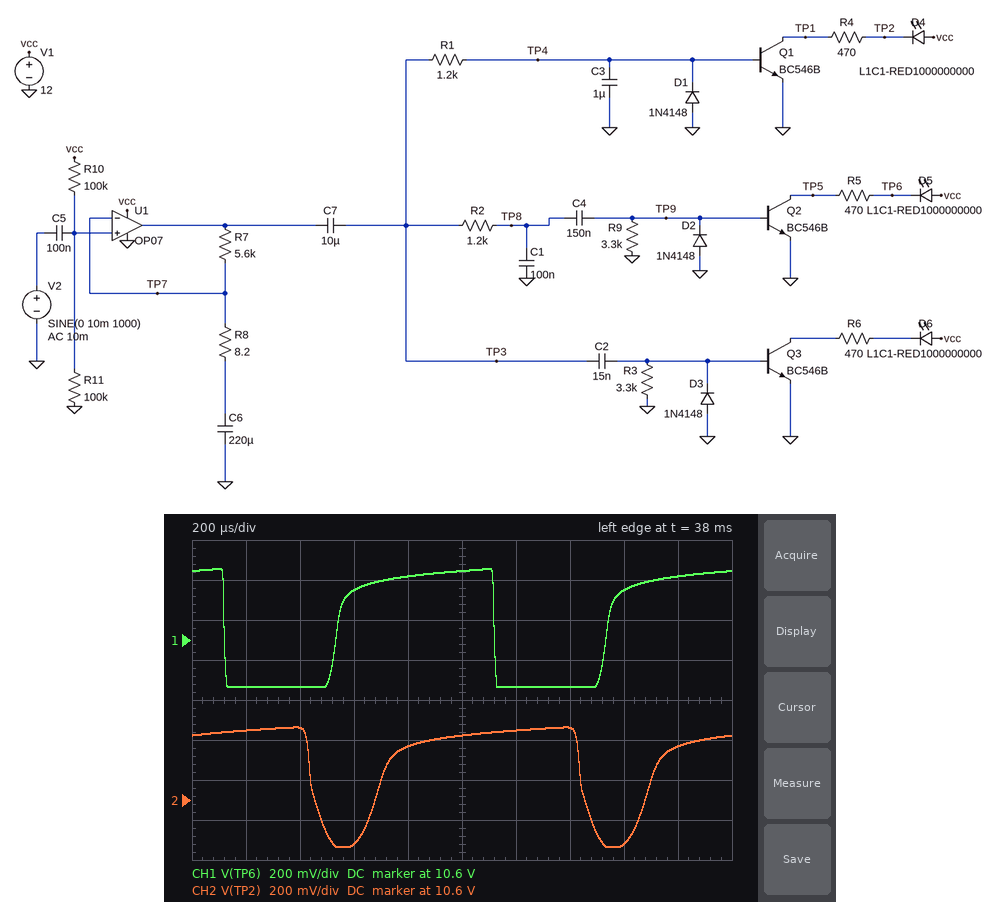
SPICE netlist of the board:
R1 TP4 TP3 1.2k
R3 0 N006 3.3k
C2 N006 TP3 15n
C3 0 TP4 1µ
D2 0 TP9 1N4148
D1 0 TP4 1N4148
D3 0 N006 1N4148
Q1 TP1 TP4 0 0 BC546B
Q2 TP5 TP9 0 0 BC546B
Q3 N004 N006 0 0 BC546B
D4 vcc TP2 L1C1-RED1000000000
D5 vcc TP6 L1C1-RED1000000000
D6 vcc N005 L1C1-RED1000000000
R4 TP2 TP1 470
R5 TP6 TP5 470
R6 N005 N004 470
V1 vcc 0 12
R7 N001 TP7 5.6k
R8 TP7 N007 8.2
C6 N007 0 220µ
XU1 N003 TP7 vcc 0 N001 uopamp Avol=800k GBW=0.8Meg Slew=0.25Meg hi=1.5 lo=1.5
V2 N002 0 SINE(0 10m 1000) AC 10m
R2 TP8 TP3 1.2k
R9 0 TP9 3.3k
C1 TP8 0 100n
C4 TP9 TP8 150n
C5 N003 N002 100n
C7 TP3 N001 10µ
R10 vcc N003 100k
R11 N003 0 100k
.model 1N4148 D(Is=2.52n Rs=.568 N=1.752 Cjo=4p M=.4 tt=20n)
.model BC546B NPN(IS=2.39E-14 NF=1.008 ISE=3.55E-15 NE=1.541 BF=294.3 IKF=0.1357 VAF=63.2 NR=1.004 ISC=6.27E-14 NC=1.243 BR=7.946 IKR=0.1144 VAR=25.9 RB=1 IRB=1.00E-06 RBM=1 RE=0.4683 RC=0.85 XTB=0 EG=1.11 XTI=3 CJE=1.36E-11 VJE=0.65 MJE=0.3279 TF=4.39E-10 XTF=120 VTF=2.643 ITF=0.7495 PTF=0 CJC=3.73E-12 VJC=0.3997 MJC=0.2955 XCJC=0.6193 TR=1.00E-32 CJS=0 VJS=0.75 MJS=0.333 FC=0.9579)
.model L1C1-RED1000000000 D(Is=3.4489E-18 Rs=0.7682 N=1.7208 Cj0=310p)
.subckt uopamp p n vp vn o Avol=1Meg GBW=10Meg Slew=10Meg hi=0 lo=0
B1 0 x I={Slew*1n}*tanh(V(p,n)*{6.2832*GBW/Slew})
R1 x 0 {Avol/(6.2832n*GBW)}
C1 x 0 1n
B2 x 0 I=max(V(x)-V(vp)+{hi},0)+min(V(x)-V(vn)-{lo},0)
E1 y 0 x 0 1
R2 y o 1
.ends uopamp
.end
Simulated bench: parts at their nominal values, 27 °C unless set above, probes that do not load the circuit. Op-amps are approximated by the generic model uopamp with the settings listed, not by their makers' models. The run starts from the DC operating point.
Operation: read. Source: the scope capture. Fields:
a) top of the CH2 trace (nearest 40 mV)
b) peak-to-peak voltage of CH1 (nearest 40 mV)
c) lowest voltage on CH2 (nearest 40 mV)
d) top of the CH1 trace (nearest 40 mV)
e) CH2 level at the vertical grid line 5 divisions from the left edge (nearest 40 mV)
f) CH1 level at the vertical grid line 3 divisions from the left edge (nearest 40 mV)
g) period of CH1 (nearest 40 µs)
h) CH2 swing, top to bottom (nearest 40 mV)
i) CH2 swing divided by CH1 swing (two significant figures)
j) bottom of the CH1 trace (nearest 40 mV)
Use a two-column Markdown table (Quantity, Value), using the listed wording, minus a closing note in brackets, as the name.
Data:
| Quantity | Value |
|---|---|
| top of the CH2 trace | 10.96 V |
| peak-to-peak voltage of CH1 | 600 mV |
| lowest voltage on CH2 | 10.36 V |
| top of the CH1 trace | 10.96 V |
| CH2 level at the vertical grid line 5 divisions from the left edge | 10.92 V |
| CH1 level at the vertical grid line 3 divisions from the left edge | 10.84 V |
| period of CH1 | 1.00 ms |
| CH2 swing, top to bottom | 600 mV |
| CH2 swing divided by CH1 swing | 1.0 |
| bottom of the CH1 trace | 10.36 V |
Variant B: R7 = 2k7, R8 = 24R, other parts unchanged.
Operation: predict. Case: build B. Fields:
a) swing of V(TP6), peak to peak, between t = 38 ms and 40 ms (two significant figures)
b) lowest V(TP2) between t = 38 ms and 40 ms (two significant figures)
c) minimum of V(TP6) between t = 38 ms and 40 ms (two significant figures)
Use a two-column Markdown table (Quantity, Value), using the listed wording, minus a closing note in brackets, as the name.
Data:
| Quantity | Value |
|---|---|
| swing of V(TP6), peak to peak, between t = 38 ms and 40 ms | 550 mV |
| lowest V(TP2) between t = 38 ms and 40 ms | 11 V |
| minimum of V(TP6) between t = 38 ms and 40 ms | 10 V |
